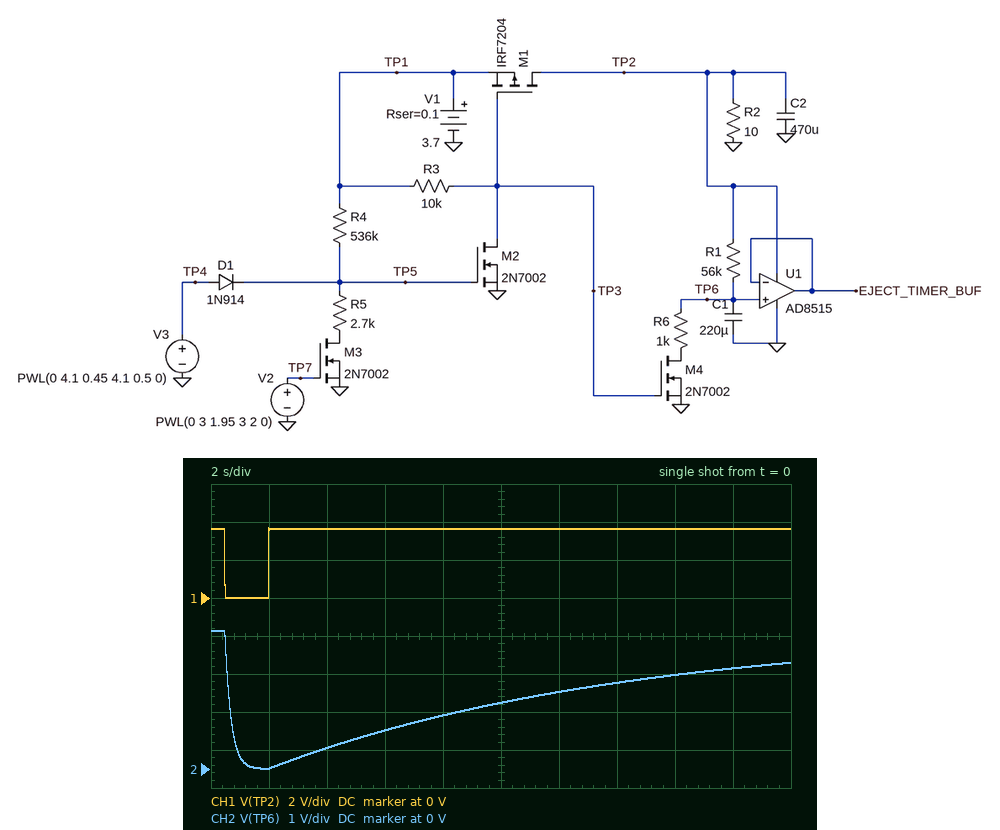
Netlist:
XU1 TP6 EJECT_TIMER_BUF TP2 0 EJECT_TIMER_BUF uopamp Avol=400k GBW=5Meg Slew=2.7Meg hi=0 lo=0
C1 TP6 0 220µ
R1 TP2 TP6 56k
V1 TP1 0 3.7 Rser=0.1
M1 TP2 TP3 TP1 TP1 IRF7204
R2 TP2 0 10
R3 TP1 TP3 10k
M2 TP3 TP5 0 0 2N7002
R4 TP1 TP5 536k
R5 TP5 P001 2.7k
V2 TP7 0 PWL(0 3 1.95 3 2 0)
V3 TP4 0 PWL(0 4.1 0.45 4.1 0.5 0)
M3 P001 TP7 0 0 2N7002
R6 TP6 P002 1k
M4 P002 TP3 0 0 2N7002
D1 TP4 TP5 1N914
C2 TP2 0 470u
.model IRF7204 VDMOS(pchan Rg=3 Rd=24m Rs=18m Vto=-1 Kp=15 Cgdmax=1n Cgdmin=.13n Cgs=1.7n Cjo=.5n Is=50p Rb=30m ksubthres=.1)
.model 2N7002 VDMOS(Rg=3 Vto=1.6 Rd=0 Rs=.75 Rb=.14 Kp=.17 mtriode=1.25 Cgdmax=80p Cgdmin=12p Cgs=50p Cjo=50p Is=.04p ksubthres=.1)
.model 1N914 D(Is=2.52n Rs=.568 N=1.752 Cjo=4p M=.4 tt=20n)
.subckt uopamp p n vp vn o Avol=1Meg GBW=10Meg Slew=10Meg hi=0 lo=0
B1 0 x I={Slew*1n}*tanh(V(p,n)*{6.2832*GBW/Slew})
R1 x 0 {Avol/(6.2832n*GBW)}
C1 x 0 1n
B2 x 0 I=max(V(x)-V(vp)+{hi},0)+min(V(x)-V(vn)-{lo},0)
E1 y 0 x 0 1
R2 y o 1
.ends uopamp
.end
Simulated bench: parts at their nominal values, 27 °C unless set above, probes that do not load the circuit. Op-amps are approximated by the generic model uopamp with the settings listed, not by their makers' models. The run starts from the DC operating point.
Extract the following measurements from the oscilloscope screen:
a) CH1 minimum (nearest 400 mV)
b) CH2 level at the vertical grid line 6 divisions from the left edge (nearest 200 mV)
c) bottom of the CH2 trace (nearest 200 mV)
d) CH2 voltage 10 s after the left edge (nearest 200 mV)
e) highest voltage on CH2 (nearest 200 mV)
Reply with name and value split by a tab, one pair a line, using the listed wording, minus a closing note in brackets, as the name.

CH1 minimum	0 V
CH2 level at the vertical grid line 6 divisions from the left edge	2.0 V
bottom of the CH2 trace	0 V
CH2 voltage 10 s after the left edge	1.8 V
highest voltage on CH2	3.6 V
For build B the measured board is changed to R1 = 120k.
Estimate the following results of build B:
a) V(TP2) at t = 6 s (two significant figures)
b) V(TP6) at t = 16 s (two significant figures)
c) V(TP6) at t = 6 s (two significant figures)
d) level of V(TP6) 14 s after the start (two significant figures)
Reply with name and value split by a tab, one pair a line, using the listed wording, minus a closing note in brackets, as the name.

V(TP2) at t = 6 s	3.6 V
V(TP6) at t = 16 s	1.5 V
V(TP6) at t = 6 s	520 mV
level of V(TP6) 14 s after the start	1.3 V
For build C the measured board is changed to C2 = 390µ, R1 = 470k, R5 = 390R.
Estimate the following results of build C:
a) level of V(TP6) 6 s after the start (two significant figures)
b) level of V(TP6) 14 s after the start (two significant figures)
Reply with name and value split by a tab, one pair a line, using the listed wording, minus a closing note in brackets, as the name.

level of V(TP6) 6 s after the start	140 mV
level of V(TP6) 14 s after the start	400 mV
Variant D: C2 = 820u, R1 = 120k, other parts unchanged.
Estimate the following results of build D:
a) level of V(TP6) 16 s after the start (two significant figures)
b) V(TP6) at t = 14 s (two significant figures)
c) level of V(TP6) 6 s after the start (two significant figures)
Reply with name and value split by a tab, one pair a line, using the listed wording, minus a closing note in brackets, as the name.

level of V(TP6) 16 s after the start	1.5 V
V(TP6) at t = 14 s	1.3 V
level of V(TP6) 6 s after the start	520 mV
